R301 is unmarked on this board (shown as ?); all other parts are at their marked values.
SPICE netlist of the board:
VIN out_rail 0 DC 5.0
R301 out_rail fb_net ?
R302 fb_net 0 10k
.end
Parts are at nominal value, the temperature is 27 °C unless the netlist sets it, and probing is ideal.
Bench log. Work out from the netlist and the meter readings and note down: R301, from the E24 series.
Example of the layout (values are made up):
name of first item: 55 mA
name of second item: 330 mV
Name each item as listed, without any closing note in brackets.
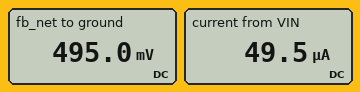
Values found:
R301, from the E24 series: 91 kΩ
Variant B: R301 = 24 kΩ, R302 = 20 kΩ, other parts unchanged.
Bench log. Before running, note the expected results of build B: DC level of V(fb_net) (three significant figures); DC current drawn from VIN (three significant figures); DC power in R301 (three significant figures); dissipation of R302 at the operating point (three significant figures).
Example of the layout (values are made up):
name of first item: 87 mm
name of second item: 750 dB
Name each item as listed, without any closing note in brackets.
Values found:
DC level of V(fb_net): 2.27 V
DC current drawn from VIN: 114 µA
DC power in R301: 310 µW
dissipation of R302 at the operating point: 258 µW
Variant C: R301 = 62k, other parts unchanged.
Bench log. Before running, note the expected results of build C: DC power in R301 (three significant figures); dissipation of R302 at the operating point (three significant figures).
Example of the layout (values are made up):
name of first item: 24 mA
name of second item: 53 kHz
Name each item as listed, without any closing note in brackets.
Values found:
DC power in R301: 299 µW
dissipation of R302 at the operating point: 48.2 µW
